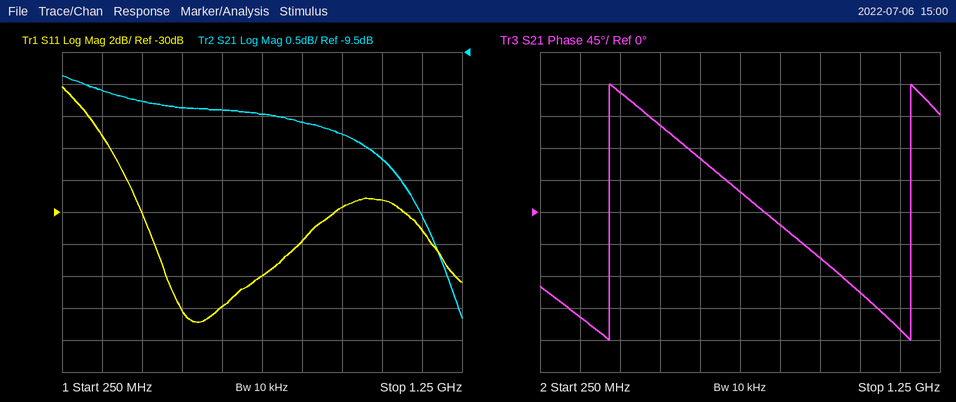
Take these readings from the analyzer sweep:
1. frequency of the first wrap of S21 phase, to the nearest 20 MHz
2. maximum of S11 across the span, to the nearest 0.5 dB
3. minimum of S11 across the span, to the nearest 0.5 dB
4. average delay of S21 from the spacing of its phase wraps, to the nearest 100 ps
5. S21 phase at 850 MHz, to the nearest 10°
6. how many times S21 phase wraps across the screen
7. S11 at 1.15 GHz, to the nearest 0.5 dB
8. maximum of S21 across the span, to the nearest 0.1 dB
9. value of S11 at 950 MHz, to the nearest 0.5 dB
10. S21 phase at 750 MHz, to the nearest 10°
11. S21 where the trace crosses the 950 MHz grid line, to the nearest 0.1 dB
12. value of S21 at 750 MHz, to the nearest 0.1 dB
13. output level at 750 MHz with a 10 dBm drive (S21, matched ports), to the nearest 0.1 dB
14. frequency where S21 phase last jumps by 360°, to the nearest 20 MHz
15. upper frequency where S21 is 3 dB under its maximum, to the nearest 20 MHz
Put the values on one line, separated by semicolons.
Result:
420 MHz; -22.0 dB; -37.0 dB; 1.3 ns; -20°; 2; -31.0 dB; -9.9 dB; -29.5 dB; 30°; -10.8 dB; -10.5 dB; -0.5 dBm; 1.18 GHz; 1.20 GHz
